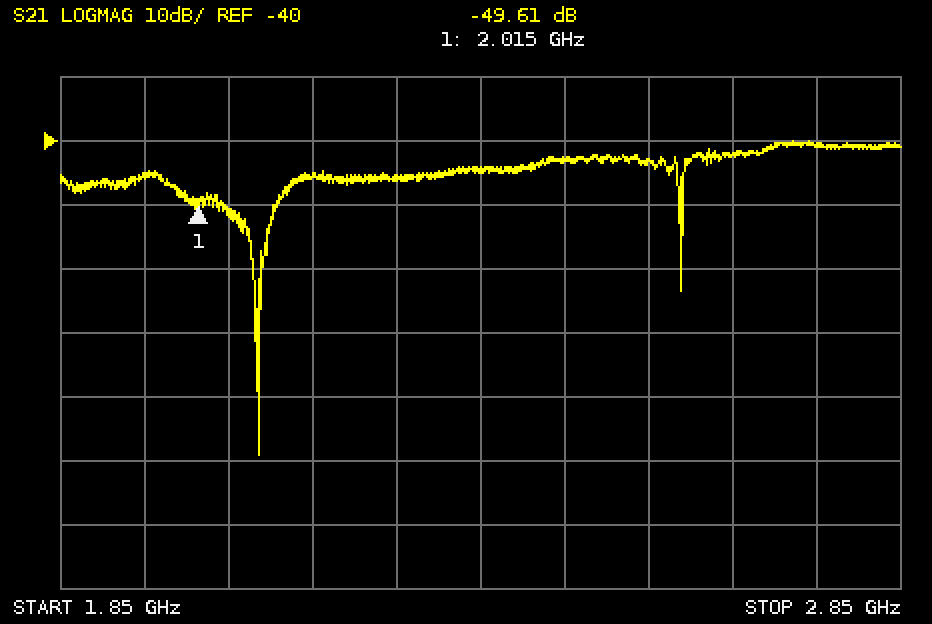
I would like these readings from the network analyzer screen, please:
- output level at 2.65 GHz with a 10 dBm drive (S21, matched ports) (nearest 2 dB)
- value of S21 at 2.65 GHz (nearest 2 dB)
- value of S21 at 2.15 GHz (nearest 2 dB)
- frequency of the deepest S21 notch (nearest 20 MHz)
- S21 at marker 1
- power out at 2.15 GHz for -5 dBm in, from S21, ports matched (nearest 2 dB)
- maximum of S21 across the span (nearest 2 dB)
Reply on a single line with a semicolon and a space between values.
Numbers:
-32 dBm; -42 dB; -46 dB; 2.08 GHz; -49.61 dB; -50 dBm; -40 dB
